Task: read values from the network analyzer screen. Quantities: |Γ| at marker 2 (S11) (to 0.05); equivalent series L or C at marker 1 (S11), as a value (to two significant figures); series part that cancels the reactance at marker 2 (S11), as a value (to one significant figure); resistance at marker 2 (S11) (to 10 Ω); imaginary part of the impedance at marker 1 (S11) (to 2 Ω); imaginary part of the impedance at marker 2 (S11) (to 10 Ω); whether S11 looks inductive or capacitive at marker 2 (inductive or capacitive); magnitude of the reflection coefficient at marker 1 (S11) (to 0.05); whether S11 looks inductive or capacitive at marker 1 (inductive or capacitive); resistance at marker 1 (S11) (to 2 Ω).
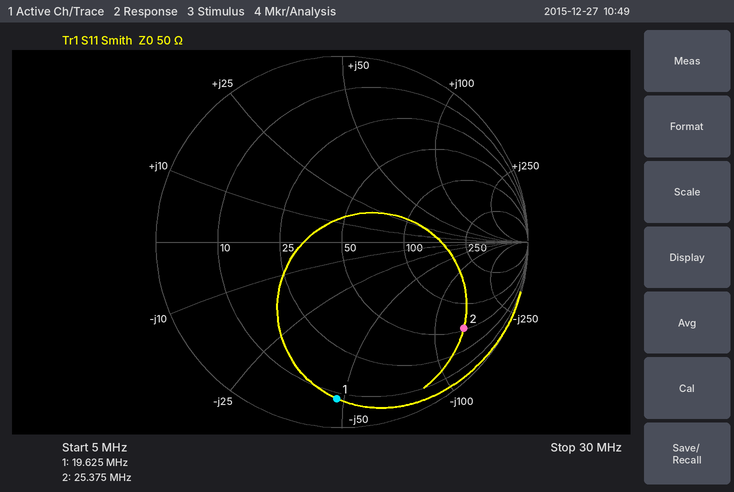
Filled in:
0.80
170 pF
900 nH
50 Ω
-48 Ω
-140 Ω
capacitive
0.85
capacitive
8 Ω
